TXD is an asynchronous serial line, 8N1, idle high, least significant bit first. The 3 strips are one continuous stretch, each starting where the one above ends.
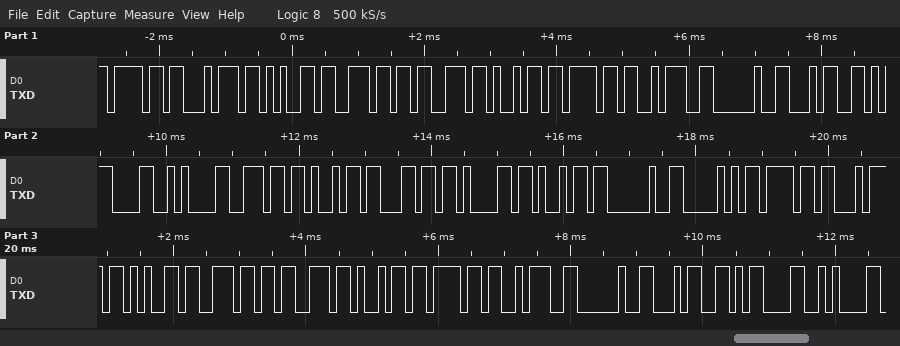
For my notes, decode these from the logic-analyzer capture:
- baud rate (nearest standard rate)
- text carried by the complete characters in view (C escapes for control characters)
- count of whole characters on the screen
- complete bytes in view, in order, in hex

9600 baud
"otensio: 4\r\nnilai Potensio: 4\r\n"
31
6F 74 65 6E 73 69 6F 3A 20 34 0D 0A 6E 69 6C 61 69 20 50 6F 74 65 6E 73 69 6F 3A 20 34 0D 0A
